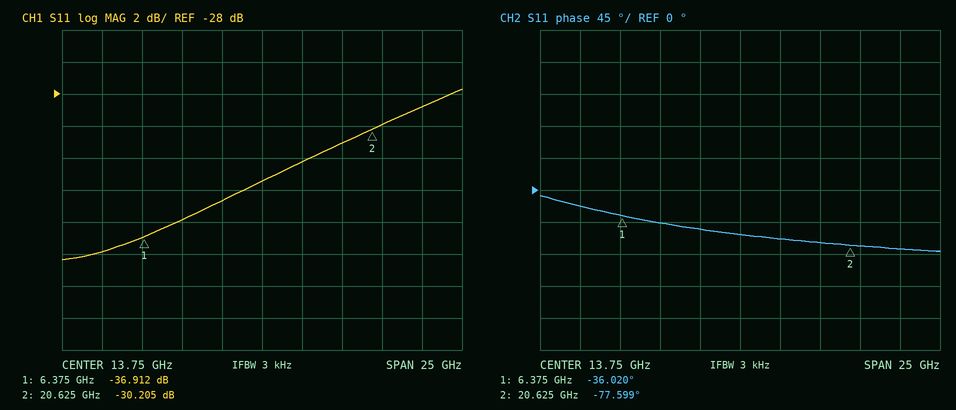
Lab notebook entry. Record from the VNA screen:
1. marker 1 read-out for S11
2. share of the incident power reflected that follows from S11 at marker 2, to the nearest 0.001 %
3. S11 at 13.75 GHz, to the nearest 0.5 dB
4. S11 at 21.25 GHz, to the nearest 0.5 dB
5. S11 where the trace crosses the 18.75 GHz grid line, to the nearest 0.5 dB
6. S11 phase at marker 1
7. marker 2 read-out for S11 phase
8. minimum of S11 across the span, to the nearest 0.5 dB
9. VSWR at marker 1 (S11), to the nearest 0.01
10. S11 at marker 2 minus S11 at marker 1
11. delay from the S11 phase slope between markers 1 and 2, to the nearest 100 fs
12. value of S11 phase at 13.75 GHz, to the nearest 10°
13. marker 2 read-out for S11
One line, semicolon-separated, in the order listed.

-36.912 dB; 0.095 %; -33.5 dB; -30.0 dB; -31.0 dB; -36.020°; -77.599°; -38.5 dB; 1.03; 6.707 dB; 8.1 ps; -60°; -30.205 dB
